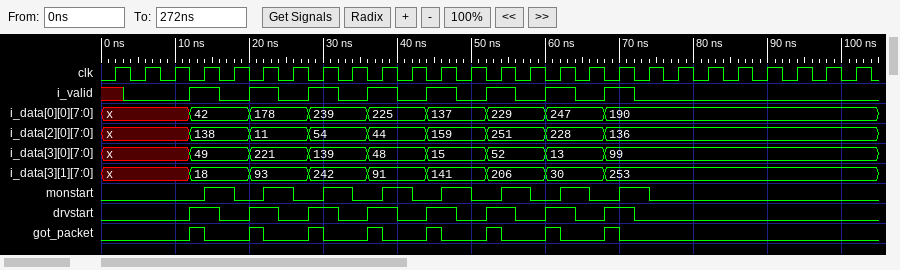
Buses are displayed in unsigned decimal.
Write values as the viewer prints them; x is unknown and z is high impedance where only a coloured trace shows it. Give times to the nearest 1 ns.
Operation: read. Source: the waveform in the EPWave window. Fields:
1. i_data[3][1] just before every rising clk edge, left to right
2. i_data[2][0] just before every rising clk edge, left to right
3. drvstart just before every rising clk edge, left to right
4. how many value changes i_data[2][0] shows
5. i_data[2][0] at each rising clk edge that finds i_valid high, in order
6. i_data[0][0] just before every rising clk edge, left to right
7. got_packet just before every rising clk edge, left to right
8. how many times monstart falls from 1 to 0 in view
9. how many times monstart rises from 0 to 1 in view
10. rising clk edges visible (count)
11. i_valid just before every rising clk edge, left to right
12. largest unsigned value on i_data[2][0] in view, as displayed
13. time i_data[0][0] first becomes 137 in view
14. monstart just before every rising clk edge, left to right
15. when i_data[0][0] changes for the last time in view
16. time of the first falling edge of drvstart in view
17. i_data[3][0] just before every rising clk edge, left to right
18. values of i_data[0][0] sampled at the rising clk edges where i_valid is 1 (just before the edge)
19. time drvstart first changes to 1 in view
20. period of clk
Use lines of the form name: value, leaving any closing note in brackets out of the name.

i_data[3][1] just before every rising clk edge, left to right: x, x, x, 18, 18, 93, 93, 242, 242, 91, 91, 141, 141, 206, 206, 30, 30, 253, 253, 253, 253, 253, 253, 253, 253, 253
i_data[2][0] just before every rising clk edge, left to right: x, x, x, 138, 138, 11, 11, 54, 54, 44, 44, 159, 159, 251, 251, 228, 228, 136, 136, 136, 136, 136, 136, 136, 136, 136
drvstart just before every rising clk edge, left to right: 0 0 0 1 0 1 0 1 0 1 0 1 0 1 0 1 0 1 0 0 0 0 0 0 0 0
how many value changes i_data[2][0] shows: 8
i_data[2][0] at each rising clk edge that finds i_valid high, in order: 138, 11, 54, 44, 159, 251, 228, 136
i_data[0][0] just before every rising clk edge, left to right: x, x, x, 42, 42, 178, 178, 239, 239, 225, 225, 137, 137, 229, 229, 247, 247, 190, 190, 190, 190, 190, 190, 190, 190, 190
got_packet just before every rising clk edge, left to right: 0 0 0 1 0 1 0 1 0 1 0 1 0 1 0 1 0 1 0 0 0 0 0 0 0 0
how many times monstart falls from 1 to 0 in view: 8
how many times monstart rises from 0 to 1 in view: 8
rising clk edges visible: 26
i_valid just before every rising clk edge, left to right: x 0 0 1 0 1 0 1 0 1 0 1 0 1 0 1 0 1 0 0 0 0 0 0 0 0
largest unsigned value on i_data[2][0] in view, as displayed: 251
time i_data[0][0] first becomes 137 in view: 44 ns
monstart just before every rising clk edge, left to right: 0 0 0 0 1 0 1 0 1 0 1 0 1 0 1 0 1 0 1 0 0 0 0 0 0 0
when i_data[0][0] changes for the last time in view: 68 ns
time of the first falling edge of drvstart in view: 16 ns
i_data[3][0] just before every rising clk edge, left to right: x, x, x, 49, 49, 221, 221, 139, 139, 48, 48, 15, 15, 52, 52, 13, 13, 99, 99, 99, 99, 99, 99, 99, 99, 99
values of i_data[0][0] sampled at the rising clk edges where i_valid is 1: 42, 178, 239, 225, 137, 229, 247, 190
time drvstart first changes to 1 in view: 12 ns
period of clk: 4 ns
